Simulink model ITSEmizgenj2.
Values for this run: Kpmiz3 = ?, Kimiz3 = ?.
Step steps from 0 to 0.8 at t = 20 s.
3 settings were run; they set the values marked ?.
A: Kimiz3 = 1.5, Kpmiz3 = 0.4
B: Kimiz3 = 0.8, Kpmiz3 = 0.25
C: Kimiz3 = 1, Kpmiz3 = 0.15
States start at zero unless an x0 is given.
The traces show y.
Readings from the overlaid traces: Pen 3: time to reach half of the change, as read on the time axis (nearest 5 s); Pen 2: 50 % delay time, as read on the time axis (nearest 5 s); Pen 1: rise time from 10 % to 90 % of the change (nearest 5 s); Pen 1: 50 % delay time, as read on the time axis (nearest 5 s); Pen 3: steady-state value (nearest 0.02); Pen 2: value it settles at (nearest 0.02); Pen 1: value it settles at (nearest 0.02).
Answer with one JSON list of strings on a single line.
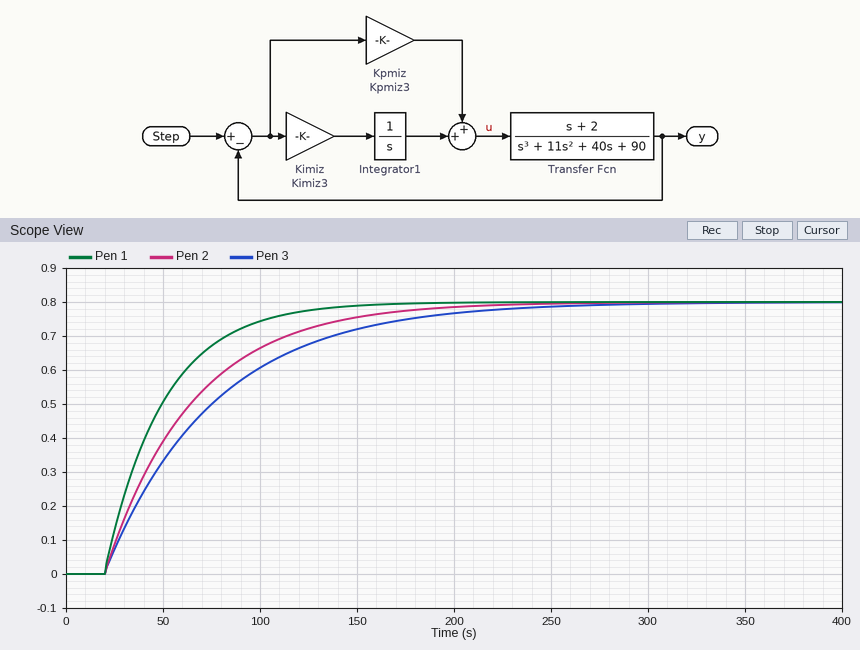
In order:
["60 s", "50 s", "65 s", "40 s", "0.80", "0.80", "0.80"]
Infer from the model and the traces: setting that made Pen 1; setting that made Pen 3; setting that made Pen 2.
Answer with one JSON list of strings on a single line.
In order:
["A", "B", "C"]
